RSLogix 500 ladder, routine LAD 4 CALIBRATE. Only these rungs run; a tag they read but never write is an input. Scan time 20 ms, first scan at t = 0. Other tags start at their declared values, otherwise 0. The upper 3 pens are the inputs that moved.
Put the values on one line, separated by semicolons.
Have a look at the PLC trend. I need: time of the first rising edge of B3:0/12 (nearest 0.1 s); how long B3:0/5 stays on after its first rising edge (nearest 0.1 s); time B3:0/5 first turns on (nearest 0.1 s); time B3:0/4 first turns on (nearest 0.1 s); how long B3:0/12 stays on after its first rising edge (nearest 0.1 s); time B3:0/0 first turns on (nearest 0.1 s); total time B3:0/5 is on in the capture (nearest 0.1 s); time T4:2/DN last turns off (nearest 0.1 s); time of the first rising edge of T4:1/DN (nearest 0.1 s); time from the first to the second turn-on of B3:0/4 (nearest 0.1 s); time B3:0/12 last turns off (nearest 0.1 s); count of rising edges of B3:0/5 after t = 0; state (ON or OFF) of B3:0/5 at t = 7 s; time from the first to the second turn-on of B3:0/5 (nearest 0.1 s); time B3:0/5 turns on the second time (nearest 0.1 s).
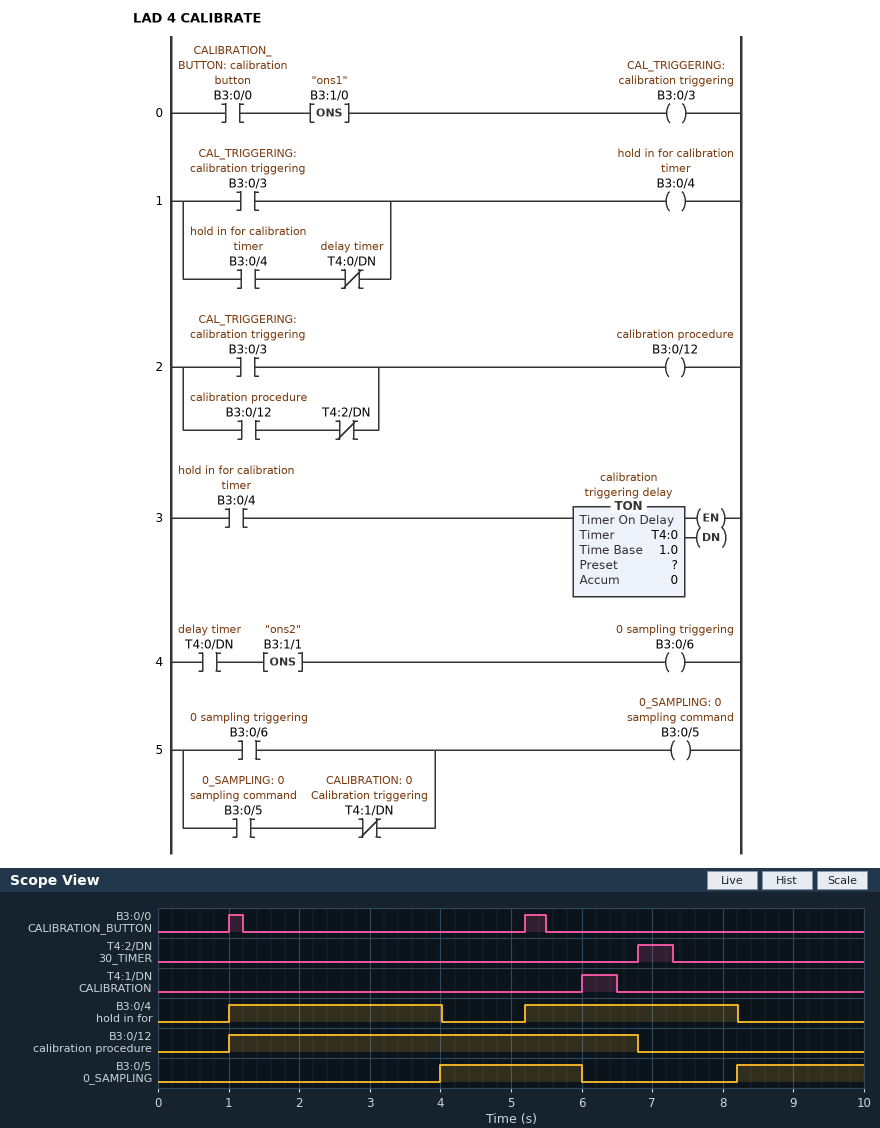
1.0 s; 2.0 s; 4.0 s; 1.0 s; 5.8 s; 1.0 s; 3.8 s; 7.3 s; 6.0 s; 4.2 s; 6.8 s; 2; OFF; 4.2 s; 8.2 s
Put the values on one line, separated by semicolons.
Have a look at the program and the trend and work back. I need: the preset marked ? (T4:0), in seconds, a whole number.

3 s
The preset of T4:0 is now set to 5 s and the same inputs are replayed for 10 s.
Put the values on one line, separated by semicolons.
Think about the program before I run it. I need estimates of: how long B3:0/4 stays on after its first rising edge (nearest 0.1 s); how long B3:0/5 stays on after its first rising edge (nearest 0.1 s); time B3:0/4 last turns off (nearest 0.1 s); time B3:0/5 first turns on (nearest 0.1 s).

5.0 s; 0.0 s; 6.0 s; 6.0 s
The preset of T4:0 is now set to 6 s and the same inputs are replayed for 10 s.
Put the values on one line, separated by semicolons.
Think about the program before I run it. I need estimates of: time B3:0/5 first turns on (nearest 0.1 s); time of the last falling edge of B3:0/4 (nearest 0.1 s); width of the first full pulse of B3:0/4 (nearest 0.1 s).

7.0 s; 7.0 s; 6.0 s
